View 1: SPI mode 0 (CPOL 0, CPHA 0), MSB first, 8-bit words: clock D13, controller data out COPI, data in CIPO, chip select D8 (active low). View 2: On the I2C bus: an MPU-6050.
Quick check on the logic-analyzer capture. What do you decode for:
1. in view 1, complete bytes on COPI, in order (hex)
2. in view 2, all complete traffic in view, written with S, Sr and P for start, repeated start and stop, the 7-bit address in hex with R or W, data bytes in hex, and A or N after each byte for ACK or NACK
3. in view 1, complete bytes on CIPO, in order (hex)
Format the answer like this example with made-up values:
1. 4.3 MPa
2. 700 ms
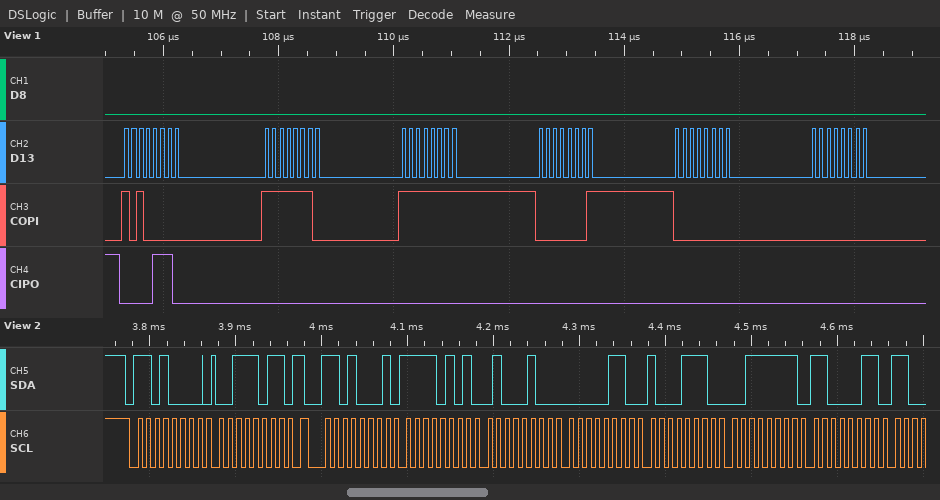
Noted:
1. A0 FE FF 01 00 00
2. S 68W A 3B A Sr 68R A F5 A 44 A 06 A 8E A 3F A C3 A
3. 0E 00 00 00 00 00
